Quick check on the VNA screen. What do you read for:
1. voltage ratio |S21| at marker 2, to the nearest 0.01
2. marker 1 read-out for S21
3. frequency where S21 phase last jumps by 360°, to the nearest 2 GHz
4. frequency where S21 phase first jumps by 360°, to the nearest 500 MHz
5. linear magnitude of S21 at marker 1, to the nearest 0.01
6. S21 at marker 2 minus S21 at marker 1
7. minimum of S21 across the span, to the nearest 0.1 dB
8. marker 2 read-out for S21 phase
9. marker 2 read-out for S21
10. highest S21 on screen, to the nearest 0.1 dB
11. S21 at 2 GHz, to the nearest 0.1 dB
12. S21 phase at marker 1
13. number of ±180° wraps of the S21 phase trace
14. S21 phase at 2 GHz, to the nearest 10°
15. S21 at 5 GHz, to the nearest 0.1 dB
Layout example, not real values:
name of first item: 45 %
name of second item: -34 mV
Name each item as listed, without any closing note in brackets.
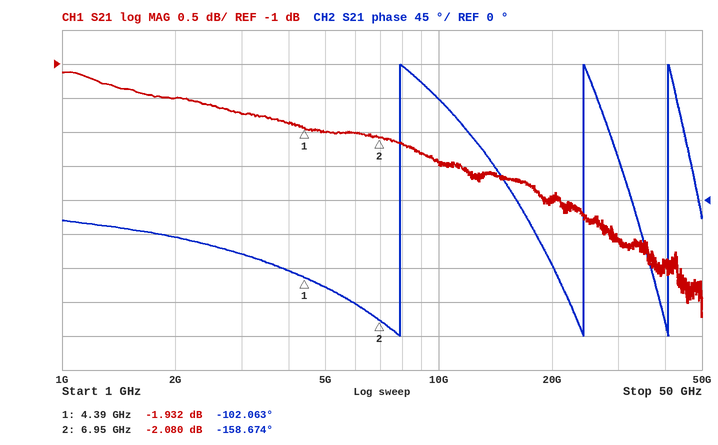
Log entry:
voltage ratio |S21| at marker 2, to the nearest 0.01: 0.79
marker 1 read-out for S21: -1.932 dB
frequency where S21 phase last jumps by 360°, to the nearest 2 GHz: 40 GHz
frequency where S21 phase first jumps by 360°, to the nearest 500 MHz: 8.0 GHz
linear magnitude of S21 at marker 1, to the nearest 0.01: 0.80
S21 at marker 2 minus S21 at marker 1: -0.148 dB
minimum of S21 across the span, to the nearest 0.1 dB: -4.7 dB
marker 2 read-out for S21 phase: -158.674°
marker 2 read-out for S21: -2.080 dB
highest S21 on screen, to the nearest 0.1 dB: -1.1 dB
S21 at 2 GHz, to the nearest 0.1 dB: -1.5 dB
S21 phase at marker 1: -102.063°
number of ±180° wraps of the S21 phase trace: 3
S21 phase at 2 GHz, to the nearest 10°: -50°
S21 at 5 GHz, to the nearest 0.1 dB: -2.0 dB
